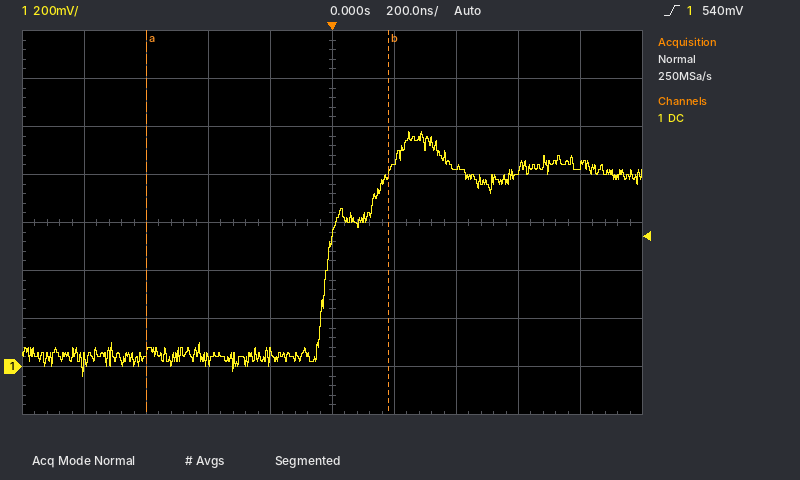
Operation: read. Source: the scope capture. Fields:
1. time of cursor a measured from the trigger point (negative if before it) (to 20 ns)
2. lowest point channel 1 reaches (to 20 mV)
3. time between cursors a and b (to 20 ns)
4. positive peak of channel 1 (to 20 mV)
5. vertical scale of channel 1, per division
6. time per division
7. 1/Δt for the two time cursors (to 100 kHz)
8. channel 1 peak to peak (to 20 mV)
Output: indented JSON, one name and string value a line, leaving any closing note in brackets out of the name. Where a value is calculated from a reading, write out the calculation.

{
  "time of cursor a measured from the trigger point (negative if before it)": "-600 ns",
  "lowest point channel 1 reaches": "-40 mV",
  "time between cursors a and b": "780 ns",
  "positive peak of channel 1": "980 mV",
  "vertical scale of channel 1, per division": "200 mV",
  "time per division": "200 ns",
  "1/Δt for the two time cursors": "1 / 780 ns ≈ 1.3 MHz",
  "channel 1 peak to peak": "980 mV − (-40 mV) = 1.02 V"
}
